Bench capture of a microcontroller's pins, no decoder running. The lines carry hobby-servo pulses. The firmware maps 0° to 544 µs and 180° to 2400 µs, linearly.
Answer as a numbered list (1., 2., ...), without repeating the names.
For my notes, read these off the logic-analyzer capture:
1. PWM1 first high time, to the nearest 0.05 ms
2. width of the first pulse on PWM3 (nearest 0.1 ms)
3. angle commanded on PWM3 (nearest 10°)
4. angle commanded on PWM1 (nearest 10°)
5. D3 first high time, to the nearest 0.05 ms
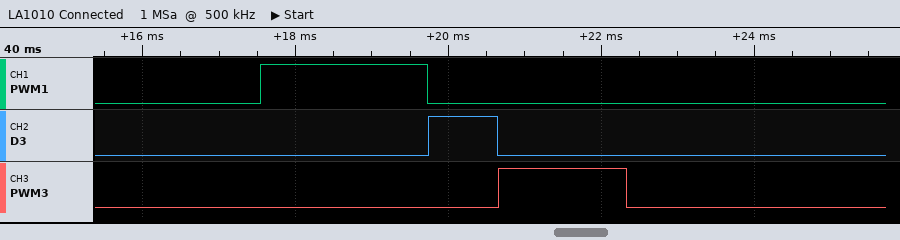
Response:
1. 2.20 ms
2. 1.7 ms
3. 110°
4. 160°
5. 0.90 ms
